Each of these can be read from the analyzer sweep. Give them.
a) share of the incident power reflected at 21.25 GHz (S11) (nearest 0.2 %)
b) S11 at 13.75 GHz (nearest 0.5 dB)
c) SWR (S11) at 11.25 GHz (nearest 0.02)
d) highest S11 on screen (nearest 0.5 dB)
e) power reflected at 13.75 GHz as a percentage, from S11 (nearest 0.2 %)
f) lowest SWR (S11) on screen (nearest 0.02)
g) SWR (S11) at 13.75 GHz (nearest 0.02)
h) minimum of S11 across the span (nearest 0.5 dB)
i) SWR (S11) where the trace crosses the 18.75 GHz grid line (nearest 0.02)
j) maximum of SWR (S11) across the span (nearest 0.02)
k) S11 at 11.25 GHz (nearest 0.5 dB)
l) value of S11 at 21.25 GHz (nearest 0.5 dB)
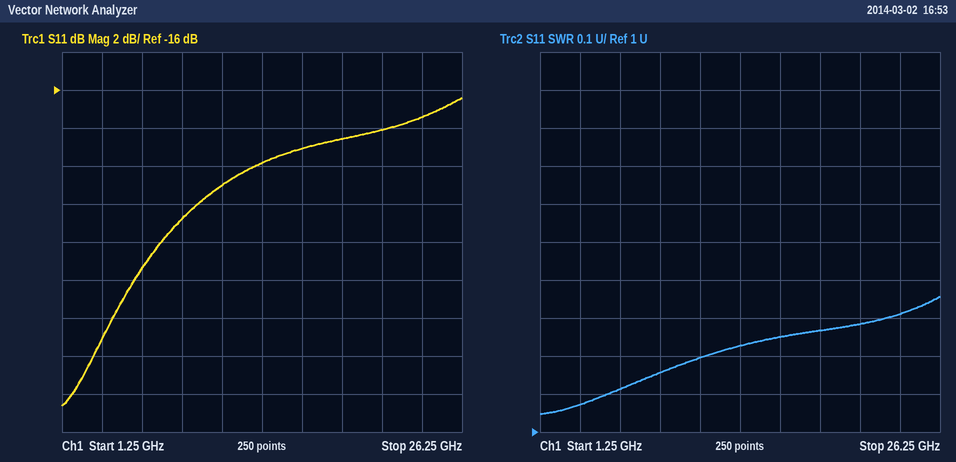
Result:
1.6 %
-20.0 dB
1.20
-16.5 dB
1.0 %
1.04
1.22
-32.5 dB
1.26
1.36
-21.0 dB
-18.0 dB
